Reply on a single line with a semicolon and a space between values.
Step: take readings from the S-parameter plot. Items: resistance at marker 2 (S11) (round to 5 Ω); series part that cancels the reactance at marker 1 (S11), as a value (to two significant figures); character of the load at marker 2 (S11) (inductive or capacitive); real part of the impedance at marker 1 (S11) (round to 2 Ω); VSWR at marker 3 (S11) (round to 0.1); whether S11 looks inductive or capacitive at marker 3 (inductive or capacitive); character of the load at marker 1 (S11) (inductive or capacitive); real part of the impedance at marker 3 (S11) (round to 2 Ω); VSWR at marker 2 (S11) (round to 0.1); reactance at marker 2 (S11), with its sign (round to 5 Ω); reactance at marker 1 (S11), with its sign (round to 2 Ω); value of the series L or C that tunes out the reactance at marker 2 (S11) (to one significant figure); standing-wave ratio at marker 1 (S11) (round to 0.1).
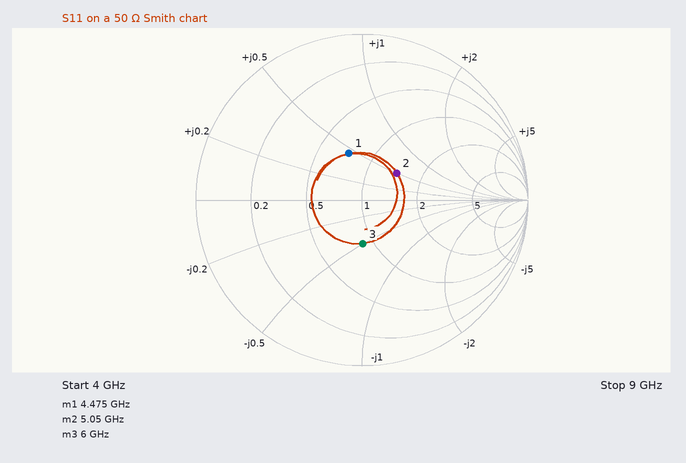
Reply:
70 Ω; 1.6 pF; inductive; 36 Ω; 1.7; capacitive; inductive; 44 Ω; 1.7; +25 Ω; +22 Ω; 1 pF; 1.8
